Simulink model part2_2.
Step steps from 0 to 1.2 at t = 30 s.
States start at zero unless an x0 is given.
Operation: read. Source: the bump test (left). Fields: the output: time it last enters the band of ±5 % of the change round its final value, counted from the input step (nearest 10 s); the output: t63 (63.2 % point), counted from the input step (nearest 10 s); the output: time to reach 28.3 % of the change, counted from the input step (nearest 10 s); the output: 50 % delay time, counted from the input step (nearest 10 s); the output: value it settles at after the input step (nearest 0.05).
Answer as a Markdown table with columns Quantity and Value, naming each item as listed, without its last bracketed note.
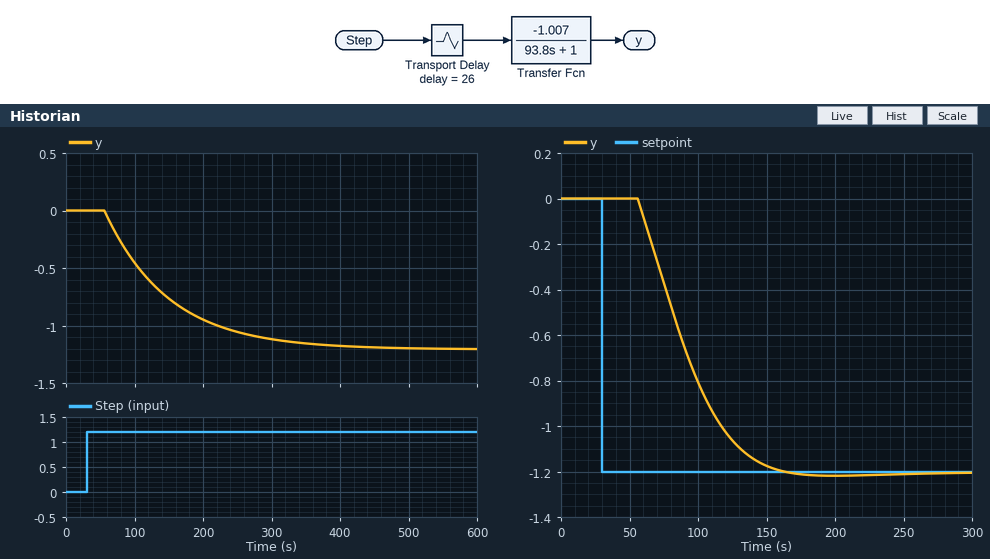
| Quantity | Value |
|---|---|
| the output: time it last enters the band of ±5 % of the change round its final value, counted from the input step | 310 s |
| the output: t63 (63.2 % point), counted from the input step | 120 s |
| the output: time to reach 28.3 % of the change, counted from the input step | 60 s |
| the output: 50 % delay time, counted from the input step | 90 s |
| the output: value it settles at after the input step | -1.20 |
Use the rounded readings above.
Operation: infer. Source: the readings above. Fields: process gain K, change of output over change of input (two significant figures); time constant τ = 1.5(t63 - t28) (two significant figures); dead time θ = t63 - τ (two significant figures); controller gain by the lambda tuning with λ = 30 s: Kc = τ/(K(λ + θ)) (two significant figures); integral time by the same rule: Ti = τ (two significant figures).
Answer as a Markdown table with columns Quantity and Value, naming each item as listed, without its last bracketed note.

| Quantity | Value |
|---|---|
| process gain K, change of output over change of input | -1.0 |
| time constant τ = 1.5(t63 - t28) | 90 s |
| dead time θ = t63 - τ | 30 s |
| controller gain by the lambda tuning with λ = 30 s: Kc = τ/(K(λ + θ)) | -1.5 |
| integral time by the same rule: Ti = τ | 90 s |
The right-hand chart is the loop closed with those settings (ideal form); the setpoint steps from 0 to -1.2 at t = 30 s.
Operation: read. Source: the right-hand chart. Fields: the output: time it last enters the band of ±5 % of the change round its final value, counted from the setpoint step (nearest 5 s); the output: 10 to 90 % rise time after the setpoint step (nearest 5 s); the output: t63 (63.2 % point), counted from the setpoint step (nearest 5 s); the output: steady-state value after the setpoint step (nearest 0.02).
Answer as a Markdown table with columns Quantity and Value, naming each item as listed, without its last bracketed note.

| Quantity | Value |
|---|---|
| the output: time it last enters the band of ±5 % of the change round its final value, counted from the setpoint step | 110 s |
| the output: 10 to 90 % rise time after the setpoint step | 65 s |
| the output: t63 (63.2 % point), counted from the setpoint step | 65 s |
| the output: steady-state value after the setpoint step | -1.20 |
